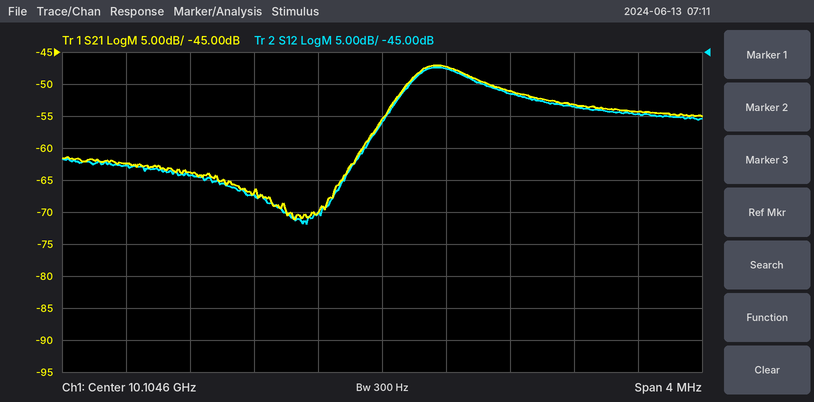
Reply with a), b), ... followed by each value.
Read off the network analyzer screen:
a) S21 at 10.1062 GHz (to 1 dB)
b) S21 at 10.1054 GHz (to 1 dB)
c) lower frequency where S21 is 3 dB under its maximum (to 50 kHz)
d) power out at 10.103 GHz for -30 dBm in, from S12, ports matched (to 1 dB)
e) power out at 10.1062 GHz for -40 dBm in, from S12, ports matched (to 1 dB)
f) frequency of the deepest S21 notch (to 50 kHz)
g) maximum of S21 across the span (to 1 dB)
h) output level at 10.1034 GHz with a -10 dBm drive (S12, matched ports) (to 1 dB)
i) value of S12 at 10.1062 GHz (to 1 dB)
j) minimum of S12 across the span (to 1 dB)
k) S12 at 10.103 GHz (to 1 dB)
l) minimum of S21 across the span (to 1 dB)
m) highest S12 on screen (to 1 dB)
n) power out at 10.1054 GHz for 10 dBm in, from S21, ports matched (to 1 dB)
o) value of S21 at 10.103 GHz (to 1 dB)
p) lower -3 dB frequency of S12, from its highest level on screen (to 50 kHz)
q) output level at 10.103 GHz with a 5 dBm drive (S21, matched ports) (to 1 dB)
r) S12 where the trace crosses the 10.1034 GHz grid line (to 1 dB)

a) -54 dB
b) -51 dB
c) 10.10475 GHz
d) -93 dBm
e) -95 dBm
f) 10.10405 GHz
g) -47 dB
h) -74 dBm
i) -55 dB
j) -72 dB
k) -63 dB
l) -71 dB
m) -47 dB
n) -41 dBm
o) -62 dB
p) 10.10475 GHz
q) -57 dBm
r) -64 dB
